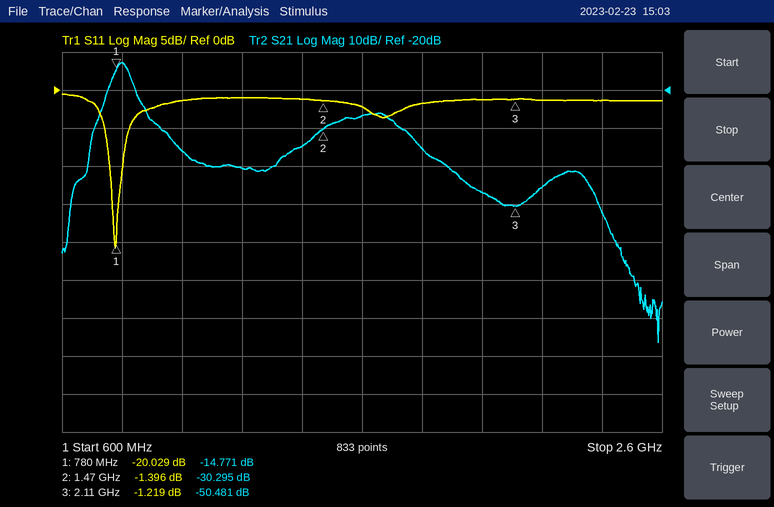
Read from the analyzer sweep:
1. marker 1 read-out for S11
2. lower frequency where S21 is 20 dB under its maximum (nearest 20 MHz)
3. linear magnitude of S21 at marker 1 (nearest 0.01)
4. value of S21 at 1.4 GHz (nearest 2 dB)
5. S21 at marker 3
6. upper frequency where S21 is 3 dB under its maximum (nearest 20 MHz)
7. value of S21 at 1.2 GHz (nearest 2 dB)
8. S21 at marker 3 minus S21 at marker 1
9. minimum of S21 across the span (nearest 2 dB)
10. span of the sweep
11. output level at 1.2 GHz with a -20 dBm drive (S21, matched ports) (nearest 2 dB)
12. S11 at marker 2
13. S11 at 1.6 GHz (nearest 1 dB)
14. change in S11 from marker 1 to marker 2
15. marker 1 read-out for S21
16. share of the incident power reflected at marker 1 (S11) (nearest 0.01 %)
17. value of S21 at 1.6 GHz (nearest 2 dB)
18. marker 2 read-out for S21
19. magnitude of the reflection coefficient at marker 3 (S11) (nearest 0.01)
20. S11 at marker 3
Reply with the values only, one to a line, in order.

-20.029 dB
700 MHz
0.18
-34 dB
-50.481 dB
820 MHz
-40 dB
-35.710 dB
-86 dB
2 GHz
-60 dBm
-1.396 dB
-2 dB
18.633 dB
-14.771 dB
0.99 %
-26 dB
-30.295 dB
0.87
-1.219 dB
